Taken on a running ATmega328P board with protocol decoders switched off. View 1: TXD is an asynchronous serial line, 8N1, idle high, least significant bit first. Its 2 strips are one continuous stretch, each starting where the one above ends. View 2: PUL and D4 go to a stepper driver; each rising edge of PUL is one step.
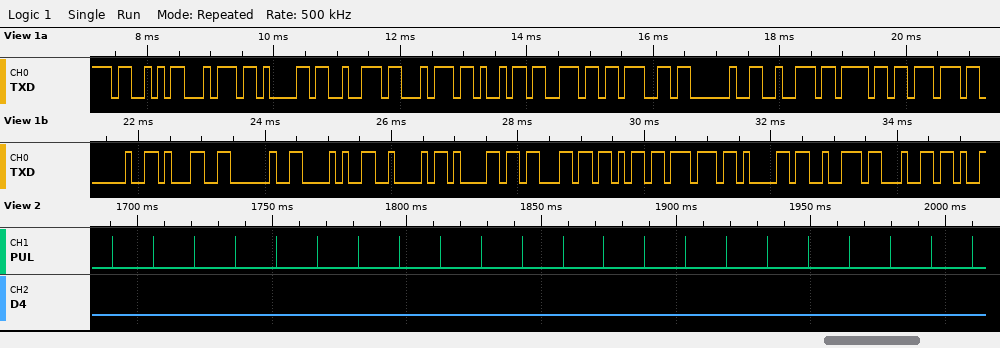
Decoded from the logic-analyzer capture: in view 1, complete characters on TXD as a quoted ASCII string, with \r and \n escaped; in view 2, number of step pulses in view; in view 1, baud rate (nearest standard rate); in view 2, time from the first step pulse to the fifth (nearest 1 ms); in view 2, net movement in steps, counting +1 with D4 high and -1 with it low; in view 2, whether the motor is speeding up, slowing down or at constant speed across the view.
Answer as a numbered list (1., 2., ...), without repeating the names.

1. "Starting row 1 (Backward"
2. 22
3. 9600 baud
4. 61 ms
5. -22
6. constant speed
